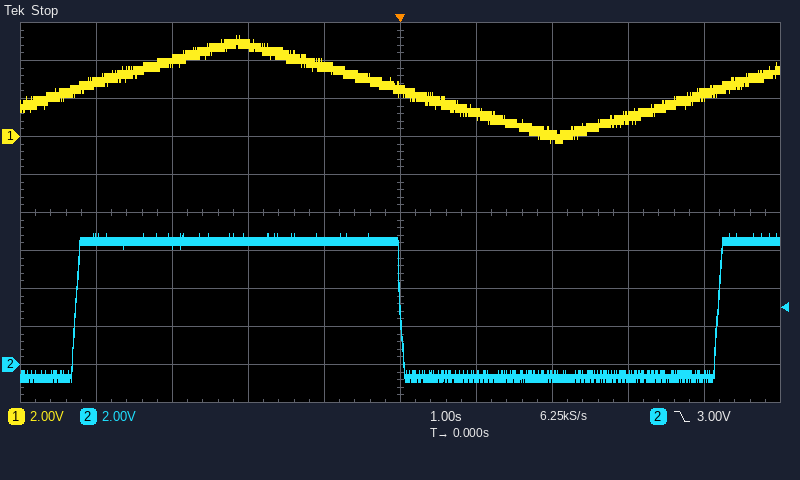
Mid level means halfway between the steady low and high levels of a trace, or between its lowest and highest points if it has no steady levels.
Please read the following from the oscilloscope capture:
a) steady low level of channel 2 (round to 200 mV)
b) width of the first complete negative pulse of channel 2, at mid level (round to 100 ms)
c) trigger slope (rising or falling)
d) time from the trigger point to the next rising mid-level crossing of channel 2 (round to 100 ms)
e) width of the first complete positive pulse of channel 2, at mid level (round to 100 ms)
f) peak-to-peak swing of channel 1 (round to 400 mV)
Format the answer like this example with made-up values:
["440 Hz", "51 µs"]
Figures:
["-600 mV", "4.2 s", "falling", "4.2 s", "4.3 s", "5.6 V"]
